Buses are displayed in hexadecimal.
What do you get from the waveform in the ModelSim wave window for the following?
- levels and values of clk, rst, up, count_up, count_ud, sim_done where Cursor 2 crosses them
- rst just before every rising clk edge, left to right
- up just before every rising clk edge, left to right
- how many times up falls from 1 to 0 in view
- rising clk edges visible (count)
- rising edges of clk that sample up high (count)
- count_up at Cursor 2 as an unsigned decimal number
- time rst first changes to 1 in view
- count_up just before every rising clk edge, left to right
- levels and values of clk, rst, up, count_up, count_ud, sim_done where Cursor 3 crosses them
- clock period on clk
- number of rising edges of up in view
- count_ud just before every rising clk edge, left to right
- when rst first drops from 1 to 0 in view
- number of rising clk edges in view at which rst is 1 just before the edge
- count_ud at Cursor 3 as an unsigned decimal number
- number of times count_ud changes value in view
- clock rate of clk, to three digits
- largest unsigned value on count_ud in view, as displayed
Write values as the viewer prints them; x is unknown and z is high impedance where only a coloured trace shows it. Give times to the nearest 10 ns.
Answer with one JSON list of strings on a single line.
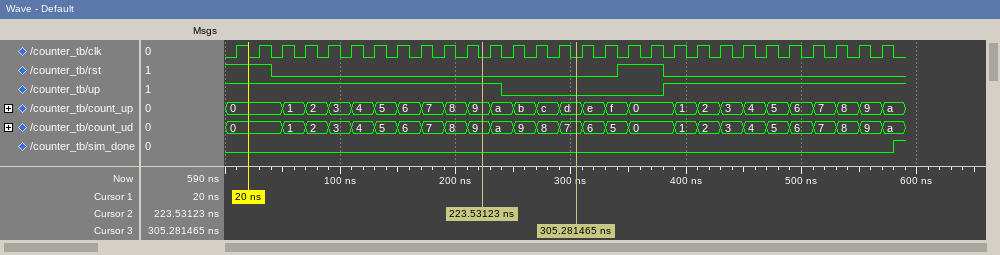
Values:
["clk=0, rst=0, up=1, count_up=9, count_ud=9, sim_done=0", "1 1 0 0 0 0 0 0 0 0 0 0 0 0 0 0 0 1 1 0 0 0 0 0 0 0 0 0 0", "1 1 1 1 1 1 1 1 1 1 1 1 0 0 0 0 0 0 0 1 1 1 1 1 1 1 1 1 1", "1", "29", "22", "9", "340 ns", "0, 0, 0, 1, 2, 3, 4, 5, 6, 7, 8, 9, a, b, c, d, e, f, 0, 0, 1, 2, 3, 4, 5, 6, 7, 8, 9", "clk=0, rst=0, up=0, count_up=d, count_ud=7, sim_done=0", "20 ns", "1", "0, 0, 0, 1, 2, 3, 4, 5, 6, 7, 8, 9, a, 9, 8, 7, 6, 5, 0, 0, 1, 2, 3, 4, 5, 6, 7, 8, 9", "40 ns", "4", "7", "26", "50.0 MHz", "a"]
